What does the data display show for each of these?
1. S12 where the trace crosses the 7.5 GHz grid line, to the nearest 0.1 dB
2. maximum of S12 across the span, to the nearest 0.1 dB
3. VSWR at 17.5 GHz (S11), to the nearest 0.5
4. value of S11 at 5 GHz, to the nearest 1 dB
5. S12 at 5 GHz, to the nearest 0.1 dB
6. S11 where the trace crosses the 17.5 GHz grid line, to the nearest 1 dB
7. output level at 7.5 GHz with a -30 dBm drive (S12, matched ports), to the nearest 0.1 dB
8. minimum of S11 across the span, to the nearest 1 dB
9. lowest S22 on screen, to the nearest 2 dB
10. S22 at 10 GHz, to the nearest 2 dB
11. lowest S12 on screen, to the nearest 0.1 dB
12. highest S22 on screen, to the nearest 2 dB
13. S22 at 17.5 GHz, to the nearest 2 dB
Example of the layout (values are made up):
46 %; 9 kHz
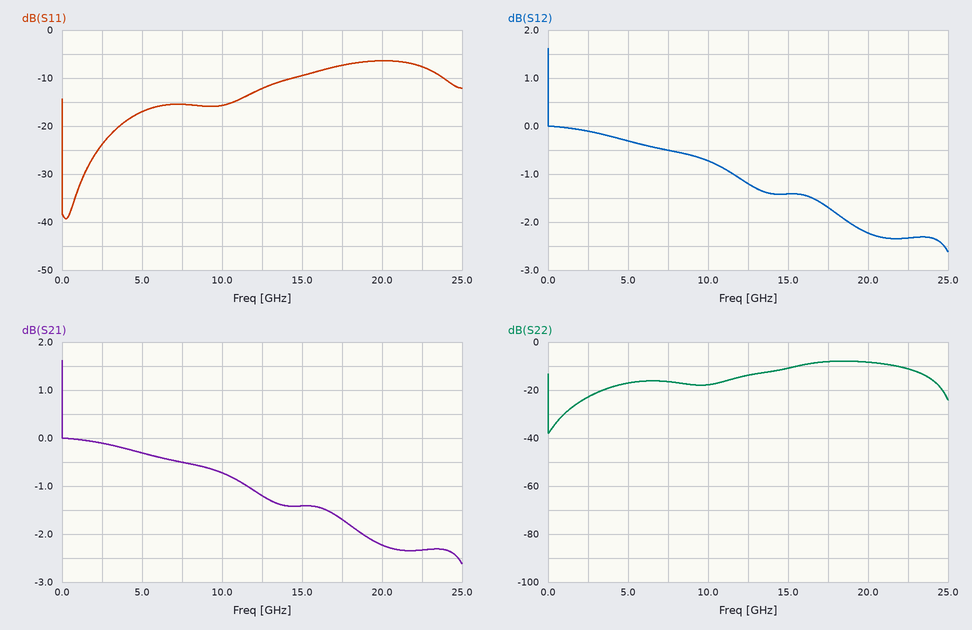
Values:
-0.5 dB; 1.6 dB; 2.5; -17 dB; -0.3 dB; -7 dB; -30.5 dBm; -39 dB; -38 dB; -18 dB; -2.6 dB; -8 dB; -8 dB
